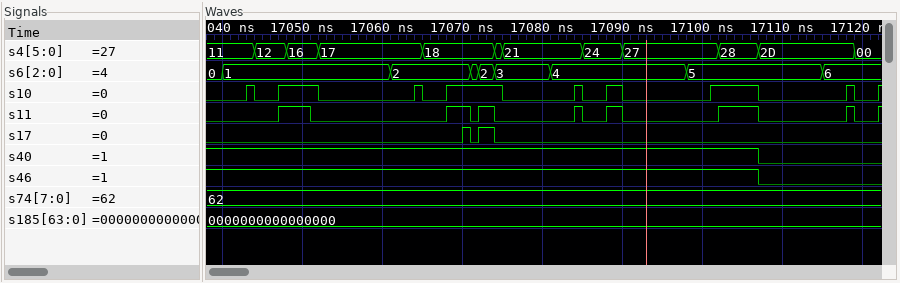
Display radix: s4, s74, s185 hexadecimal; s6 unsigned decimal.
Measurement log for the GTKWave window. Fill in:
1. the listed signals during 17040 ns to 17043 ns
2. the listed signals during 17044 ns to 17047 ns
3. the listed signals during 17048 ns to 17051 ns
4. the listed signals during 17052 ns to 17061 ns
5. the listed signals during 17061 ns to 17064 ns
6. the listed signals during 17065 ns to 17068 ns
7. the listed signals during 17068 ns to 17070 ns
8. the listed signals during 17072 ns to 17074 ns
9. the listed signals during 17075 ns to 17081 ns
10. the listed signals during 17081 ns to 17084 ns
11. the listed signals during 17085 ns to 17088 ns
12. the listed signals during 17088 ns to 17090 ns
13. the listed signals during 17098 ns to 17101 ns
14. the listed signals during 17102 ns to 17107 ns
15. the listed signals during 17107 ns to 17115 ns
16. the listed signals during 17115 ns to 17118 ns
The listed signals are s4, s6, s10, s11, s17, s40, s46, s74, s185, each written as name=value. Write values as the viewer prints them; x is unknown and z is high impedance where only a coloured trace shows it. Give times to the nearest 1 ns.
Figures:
s4=11, s6=1, s10=0, s11=0, s17=0, s40=1, s46=1, s74=62, s185=0000000000000000
s4=12, s6=1, s10=0, s11=0, s17=0, s40=1, s46=1, s74=62, s185=0000000000000000
s4=16, s6=1, s10=1, s11=1, s17=0, s40=1, s46=1, s74=62, s185=0000000000000000
s4=17, s6=1, s10=0, s11=0, s17=0, s40=1, s46=1, s74=62, s185=0000000000000000
s4=17, s6=2, s10=0, s11=0, s17=0, s40=1, s46=1, s74=62, s185=0000000000000000
s4=18, s6=2, s10=0, s11=0, s17=0, s40=1, s46=1, s74=62, s185=0000000000000000
s4=18, s6=2, s10=1, s11=1, s17=0, s40=1, s46=1, s74=62, s185=0000000000000000
s4=18, s6=2, s10=1, s11=1, s17=1, s40=1, s46=1, s74=62, s185=0000000000000000
s4=21, s6=3, s10=0, s11=0, s17=0, s40=1, s46=1, s74=62, s185=0000000000000000
s4=21, s6=4, s10=0, s11=0, s17=0, s40=1, s46=1, s74=62, s185=0000000000000000
s4=24, s6=4, s10=0, s11=0, s17=0, s40=1, s46=1, s74=62, s185=0000000000000000
s4=24, s6=4, s10=1, s11=1, s17=0, s40=1, s46=1, s74=62, s185=0000000000000000
s4=27, s6=5, s10=0, s11=0, s17=0, s40=1, s46=1, s74=62, s185=0000000000000000
s4=28, s6=5, s10=1, s11=1, s17=0, s40=1, s46=1, s74=62, s185=0000000000000000
s4=2D, s6=5, s10=0, s11=0, s17=0, s40=0, s46=0, s74=62, s185=0000000000000000
s4=2D, s6=6, s10=0, s11=0, s17=0, s40=0, s46=0, s74=62, s185=0000000000000000
